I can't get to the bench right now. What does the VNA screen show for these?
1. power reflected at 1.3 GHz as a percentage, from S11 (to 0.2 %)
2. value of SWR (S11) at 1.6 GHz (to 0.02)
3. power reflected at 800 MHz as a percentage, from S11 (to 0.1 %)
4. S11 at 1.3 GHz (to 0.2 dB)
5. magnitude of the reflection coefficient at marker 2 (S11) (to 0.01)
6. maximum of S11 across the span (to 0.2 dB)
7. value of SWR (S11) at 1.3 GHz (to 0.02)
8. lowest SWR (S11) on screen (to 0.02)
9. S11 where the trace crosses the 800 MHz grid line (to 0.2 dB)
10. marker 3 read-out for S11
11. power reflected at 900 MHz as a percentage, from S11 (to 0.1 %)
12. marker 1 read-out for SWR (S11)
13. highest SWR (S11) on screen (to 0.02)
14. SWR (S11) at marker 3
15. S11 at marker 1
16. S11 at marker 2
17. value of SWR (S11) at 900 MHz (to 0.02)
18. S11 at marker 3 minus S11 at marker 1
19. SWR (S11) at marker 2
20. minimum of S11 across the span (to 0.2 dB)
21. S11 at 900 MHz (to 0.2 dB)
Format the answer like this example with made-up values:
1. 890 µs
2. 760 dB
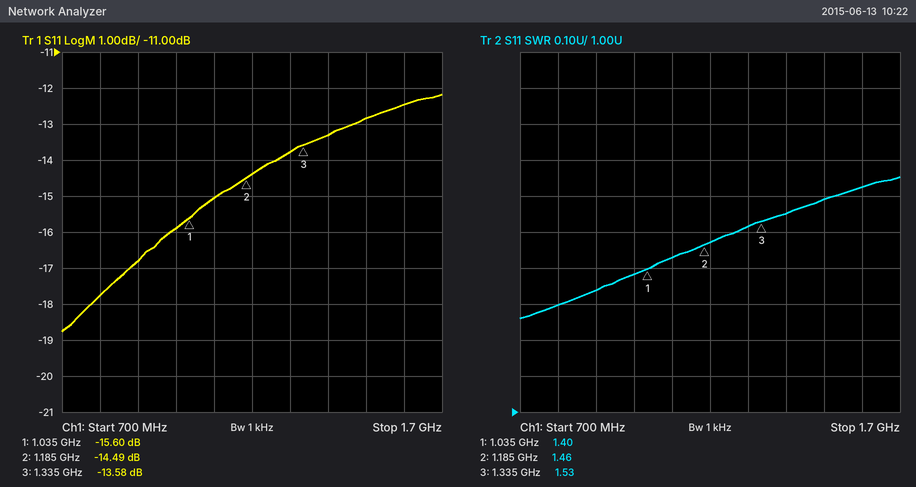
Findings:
1. 4.2 %
2. 1.62
3. 1.7 %
4. -13.8 dB
5. 0.19
6. -12.2 dB
7. 1.52
8. 1.26
9. -17.8 dB
10. -13.58 dB
11. 2.1 %
12. 1.40
13. 1.66
14. 1.53
15. -15.60 dB
16. -14.49 dB
17. 1.34
18. 2.02 dB
19. 1.46
20. -18.8 dB
21. -16.8 dB
